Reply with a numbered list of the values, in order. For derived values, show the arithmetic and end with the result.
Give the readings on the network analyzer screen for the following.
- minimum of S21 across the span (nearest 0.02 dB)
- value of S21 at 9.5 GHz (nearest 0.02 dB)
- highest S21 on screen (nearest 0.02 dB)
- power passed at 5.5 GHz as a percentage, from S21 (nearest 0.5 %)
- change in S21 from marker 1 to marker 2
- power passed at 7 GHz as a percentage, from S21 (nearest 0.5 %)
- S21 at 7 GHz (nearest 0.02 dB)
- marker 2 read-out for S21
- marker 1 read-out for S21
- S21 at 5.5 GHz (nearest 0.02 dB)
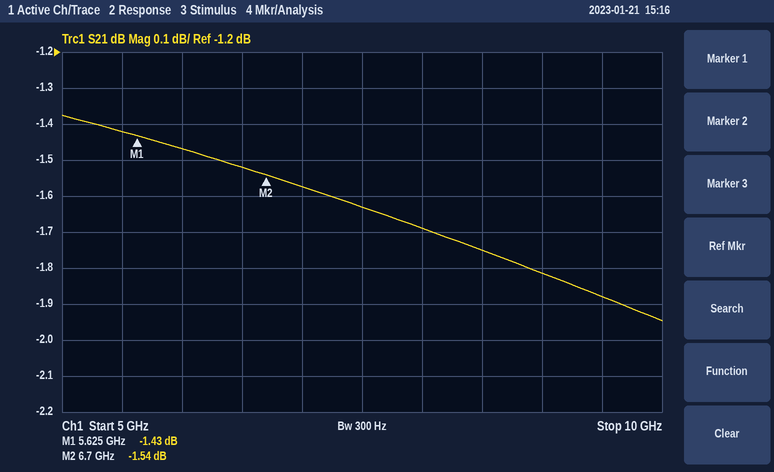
1. -1.94 dB
2. -1.88 dB
3. -1.38 dB
4. 10^(-1.42/10) ≈ 72.1 %, so 72.0 % to the nearest 0.5 %
5. -1.54 − (-1.43) = -0.11 dB
6. 10^(-1.58/10) ≈ 69.5 %
7. -1.58 dB
8. -1.54 dB
9. -1.43 dB
10. -1.42 dB
